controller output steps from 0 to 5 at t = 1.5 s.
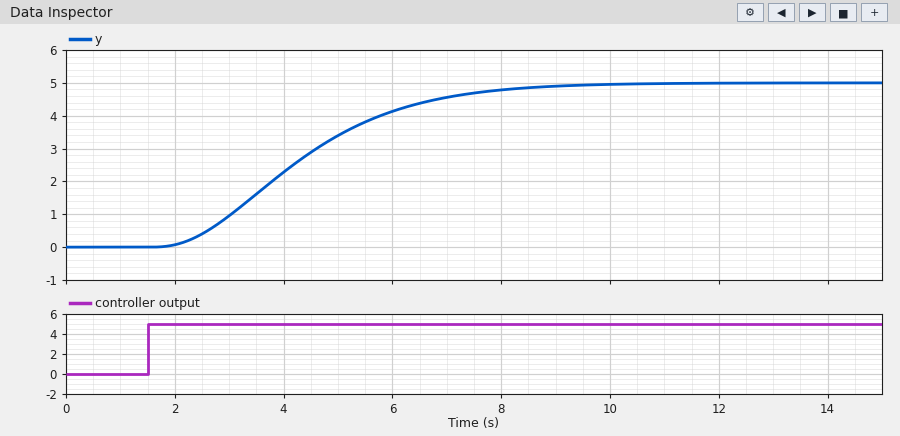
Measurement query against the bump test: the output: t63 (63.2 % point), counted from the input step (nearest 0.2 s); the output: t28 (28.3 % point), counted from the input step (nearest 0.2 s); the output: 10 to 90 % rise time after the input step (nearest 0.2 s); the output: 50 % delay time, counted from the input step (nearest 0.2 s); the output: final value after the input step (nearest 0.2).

3.2 s
1.8 s
4.2 s
2.6 s
5.0
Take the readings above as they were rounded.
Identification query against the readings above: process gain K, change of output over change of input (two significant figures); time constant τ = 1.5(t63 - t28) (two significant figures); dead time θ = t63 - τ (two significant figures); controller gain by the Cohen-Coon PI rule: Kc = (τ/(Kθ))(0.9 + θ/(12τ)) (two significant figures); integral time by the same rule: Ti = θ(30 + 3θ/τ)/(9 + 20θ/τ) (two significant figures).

1.0
2.1 s
1.1 s
1.8
1.8 s
